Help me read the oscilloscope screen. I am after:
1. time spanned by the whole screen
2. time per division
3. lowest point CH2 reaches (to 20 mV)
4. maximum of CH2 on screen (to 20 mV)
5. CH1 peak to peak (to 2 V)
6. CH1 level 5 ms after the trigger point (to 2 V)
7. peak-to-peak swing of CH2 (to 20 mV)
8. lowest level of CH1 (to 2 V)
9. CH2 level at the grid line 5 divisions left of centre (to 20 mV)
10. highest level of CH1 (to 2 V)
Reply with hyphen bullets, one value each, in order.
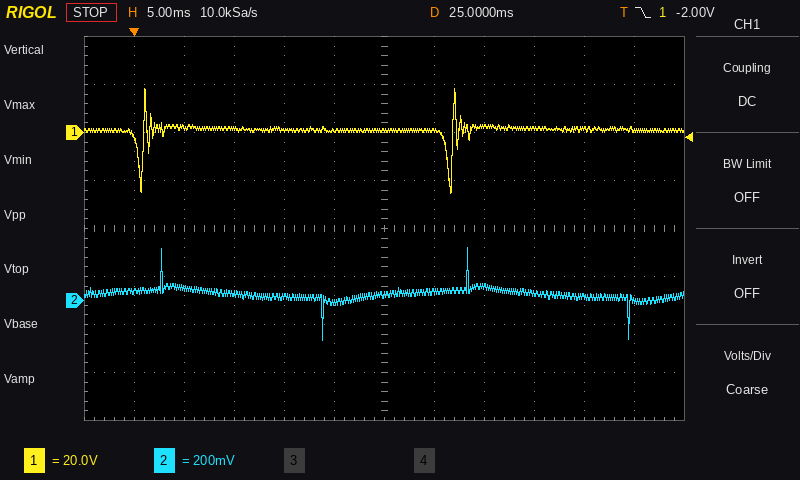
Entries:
- 60 ms
- 5 ms
- -160 mV
- 220 mV
- 44 V
- 2 V
- 380 mV
- -26 V
- 40 mV
- 18 V
